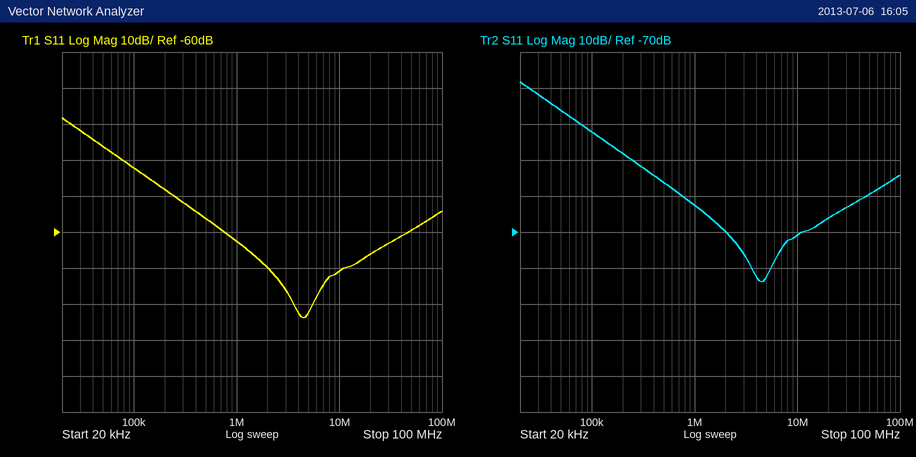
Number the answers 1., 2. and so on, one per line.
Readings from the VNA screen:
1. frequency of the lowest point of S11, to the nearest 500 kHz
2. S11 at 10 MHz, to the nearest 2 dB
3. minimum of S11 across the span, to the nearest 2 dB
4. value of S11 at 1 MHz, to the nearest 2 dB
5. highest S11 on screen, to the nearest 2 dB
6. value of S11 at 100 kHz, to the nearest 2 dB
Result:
1. 4.5 MHz
2. -70 dB
3. -84 dB
4. -62 dB
5. -28 dB
6. -42 dB
